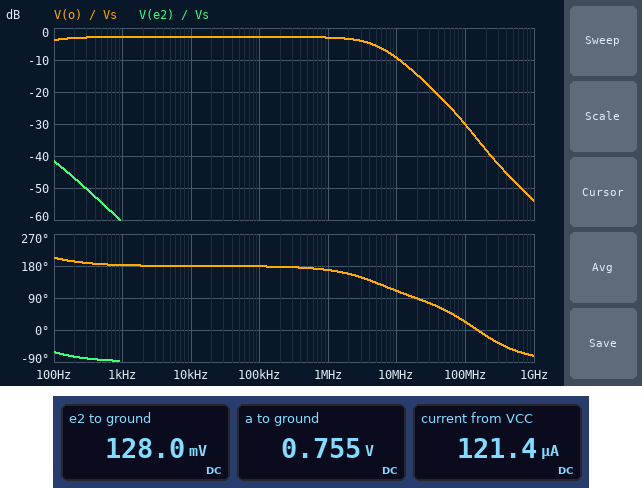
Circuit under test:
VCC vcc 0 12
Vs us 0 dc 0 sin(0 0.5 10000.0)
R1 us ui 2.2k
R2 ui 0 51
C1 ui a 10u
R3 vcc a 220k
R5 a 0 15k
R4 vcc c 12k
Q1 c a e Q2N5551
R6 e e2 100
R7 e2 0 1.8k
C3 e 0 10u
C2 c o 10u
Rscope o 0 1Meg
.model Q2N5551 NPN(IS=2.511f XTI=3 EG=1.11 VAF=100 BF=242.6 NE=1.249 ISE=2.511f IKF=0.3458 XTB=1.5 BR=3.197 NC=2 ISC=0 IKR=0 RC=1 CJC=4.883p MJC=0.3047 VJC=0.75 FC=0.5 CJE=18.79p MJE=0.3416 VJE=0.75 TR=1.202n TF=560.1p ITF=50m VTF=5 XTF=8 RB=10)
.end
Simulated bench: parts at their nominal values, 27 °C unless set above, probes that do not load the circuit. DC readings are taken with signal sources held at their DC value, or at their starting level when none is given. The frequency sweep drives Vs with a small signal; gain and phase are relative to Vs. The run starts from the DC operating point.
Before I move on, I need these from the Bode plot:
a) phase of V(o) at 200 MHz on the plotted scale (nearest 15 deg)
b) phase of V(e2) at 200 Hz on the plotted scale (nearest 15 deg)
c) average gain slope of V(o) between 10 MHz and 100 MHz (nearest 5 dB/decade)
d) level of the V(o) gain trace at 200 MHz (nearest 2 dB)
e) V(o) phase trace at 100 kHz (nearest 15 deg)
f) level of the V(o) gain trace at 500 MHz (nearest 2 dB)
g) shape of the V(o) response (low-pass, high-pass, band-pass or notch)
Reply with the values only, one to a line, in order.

-15 deg
-75 deg
-20 dB/decade
-38 dB
180 deg
-48 dB
low-pass
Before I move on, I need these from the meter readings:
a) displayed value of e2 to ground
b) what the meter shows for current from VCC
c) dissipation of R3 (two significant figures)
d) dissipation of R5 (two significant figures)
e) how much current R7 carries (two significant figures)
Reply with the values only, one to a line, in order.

128.0 mV
121.4 µA
570 µW
38 µW
71 µA
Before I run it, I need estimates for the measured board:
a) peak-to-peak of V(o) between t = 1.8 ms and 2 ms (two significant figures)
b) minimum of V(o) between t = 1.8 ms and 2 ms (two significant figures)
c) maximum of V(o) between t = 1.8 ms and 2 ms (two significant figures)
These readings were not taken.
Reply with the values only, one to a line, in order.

730 mV
-430 mV
300 mV
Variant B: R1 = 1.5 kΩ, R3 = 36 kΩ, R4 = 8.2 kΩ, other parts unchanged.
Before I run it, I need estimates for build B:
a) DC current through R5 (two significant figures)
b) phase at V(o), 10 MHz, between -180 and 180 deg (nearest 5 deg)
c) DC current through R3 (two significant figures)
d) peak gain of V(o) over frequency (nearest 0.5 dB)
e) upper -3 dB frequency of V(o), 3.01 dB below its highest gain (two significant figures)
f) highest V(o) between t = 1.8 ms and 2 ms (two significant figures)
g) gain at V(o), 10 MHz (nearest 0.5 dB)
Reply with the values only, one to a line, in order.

200 µA
155 deg
250 µA
-17.0 dB
25 MHz
2.5 V
-17.5 dB
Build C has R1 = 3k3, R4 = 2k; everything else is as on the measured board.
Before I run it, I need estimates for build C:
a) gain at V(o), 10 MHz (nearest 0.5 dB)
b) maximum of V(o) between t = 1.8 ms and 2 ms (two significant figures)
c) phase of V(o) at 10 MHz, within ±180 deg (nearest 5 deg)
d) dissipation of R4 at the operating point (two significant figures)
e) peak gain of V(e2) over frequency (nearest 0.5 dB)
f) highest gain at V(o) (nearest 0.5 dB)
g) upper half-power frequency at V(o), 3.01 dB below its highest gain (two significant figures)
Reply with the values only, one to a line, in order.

-22.0 dB
37 mV
155 deg
9.9 µW
-38.5 dB
-21.5 dB
28 MHz
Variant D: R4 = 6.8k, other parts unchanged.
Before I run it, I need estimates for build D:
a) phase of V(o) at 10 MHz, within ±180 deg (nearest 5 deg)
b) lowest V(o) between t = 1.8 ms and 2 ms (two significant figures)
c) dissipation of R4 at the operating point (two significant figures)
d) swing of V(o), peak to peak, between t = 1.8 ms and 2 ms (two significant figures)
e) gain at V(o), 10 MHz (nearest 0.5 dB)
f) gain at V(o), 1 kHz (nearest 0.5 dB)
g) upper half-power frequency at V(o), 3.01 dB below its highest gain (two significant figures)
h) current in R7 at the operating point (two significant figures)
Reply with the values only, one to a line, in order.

125 deg
-240 mV
34 µW
420 mV
-11.0 dB
-7.5 dB
9.3 MHz
71 µA
